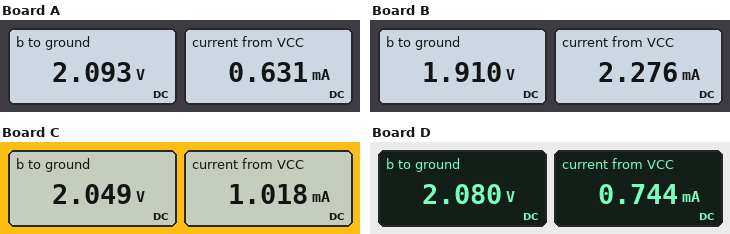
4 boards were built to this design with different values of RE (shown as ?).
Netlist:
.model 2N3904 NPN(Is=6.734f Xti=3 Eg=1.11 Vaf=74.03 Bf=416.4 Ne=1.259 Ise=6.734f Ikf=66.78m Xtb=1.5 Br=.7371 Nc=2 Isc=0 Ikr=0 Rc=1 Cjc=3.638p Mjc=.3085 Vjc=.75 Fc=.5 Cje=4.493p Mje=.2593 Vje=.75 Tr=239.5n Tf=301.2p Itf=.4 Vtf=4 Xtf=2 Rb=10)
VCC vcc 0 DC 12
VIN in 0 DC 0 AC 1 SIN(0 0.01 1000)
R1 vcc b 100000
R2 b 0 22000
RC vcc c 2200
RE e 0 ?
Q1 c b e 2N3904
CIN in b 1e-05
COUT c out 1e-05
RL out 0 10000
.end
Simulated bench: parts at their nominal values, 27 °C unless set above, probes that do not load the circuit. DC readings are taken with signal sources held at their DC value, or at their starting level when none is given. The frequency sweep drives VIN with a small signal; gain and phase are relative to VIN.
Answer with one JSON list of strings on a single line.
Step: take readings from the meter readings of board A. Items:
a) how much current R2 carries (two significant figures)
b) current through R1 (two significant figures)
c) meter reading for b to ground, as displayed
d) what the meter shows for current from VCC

["95 µA", "99 µA", "2.093 V", "0.631 mA"]
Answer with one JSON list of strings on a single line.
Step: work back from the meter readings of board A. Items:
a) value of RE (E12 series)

["2.7 kΩ"]
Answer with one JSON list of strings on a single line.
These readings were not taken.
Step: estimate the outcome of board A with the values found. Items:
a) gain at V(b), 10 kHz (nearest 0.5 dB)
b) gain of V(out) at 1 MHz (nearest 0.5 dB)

["0 dB", "-3.5 dB"]
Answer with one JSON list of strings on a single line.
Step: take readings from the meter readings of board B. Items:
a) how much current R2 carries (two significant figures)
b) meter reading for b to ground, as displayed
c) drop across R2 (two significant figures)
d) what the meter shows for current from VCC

["87 µA", "1.910 V", "1.9 V", "2.276 mA"]
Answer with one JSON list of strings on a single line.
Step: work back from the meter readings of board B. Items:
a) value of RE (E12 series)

["560 Ω"]
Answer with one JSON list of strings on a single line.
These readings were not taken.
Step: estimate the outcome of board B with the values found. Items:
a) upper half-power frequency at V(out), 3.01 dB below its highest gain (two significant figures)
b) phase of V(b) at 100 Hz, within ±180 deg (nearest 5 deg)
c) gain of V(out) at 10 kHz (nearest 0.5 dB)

["54 MHz", "0 deg", "10.0 dB"]
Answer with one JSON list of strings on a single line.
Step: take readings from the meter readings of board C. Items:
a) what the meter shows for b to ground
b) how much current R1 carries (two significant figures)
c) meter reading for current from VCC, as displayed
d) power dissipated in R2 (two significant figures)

["2.049 V", "100 µA", "1.018 mA", "190 µW"]
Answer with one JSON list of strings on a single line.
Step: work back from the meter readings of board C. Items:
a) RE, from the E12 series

["1.5 kΩ"]
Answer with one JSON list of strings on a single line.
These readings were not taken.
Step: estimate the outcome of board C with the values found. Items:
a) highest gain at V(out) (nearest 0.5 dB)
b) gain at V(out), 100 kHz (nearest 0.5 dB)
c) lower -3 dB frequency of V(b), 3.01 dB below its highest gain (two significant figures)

["1.5 dB", "1.5 dB", "950 mHz"]
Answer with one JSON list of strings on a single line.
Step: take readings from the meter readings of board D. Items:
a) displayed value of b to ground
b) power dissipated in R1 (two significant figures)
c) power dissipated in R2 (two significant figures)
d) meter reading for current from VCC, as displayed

["2.080 V", "980 µW", "200 µW", "0.744 mA"]
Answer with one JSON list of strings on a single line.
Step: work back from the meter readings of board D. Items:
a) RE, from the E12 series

["2.2 kΩ"]
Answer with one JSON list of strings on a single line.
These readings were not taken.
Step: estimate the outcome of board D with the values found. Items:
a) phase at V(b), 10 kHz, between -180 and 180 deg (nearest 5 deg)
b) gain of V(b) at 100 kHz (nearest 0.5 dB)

["0 deg", "0 dB"]
